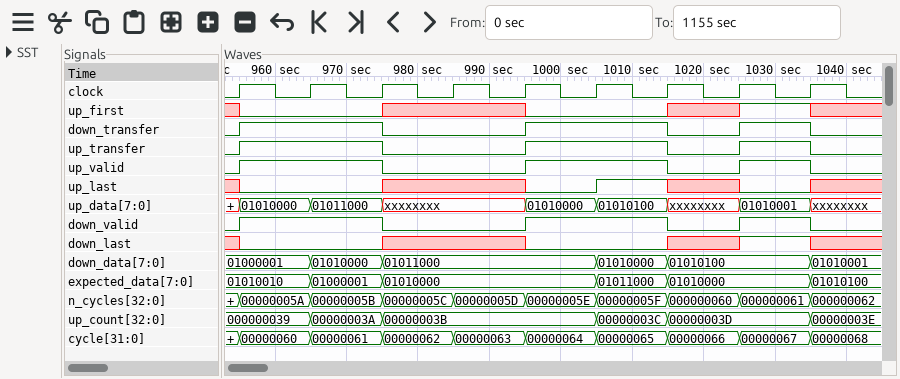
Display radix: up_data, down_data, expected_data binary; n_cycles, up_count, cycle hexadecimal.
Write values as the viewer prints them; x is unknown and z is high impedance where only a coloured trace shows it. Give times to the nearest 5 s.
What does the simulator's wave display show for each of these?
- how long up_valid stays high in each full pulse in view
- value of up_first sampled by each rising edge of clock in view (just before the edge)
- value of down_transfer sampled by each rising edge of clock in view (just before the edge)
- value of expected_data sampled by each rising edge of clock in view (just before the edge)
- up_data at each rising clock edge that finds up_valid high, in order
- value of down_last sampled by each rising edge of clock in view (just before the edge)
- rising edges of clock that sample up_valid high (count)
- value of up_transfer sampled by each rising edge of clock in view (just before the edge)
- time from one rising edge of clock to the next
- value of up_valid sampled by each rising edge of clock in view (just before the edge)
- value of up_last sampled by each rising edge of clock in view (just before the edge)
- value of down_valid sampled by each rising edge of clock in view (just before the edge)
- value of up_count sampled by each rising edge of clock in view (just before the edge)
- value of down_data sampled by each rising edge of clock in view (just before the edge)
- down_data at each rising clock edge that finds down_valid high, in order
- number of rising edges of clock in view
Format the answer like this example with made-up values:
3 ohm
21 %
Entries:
20 s, 20 s, 10 s
x 0 0 x x 0 0 x 1
0 1 1 0 0 1 1 0 1
01010010, 01010010, 01000001, 01010000, 01010000, 01010000, 01011000, 01010000, 01010000
01010000, 01011000, 01010000, 01010100, 01010001
x 0 0 x x 0 0 x 1
5
0 1 1 0 0 1 1 0 1
10 s
0 1 1 0 0 1 1 0 1
x 0 0 x x 0 1 x 0
0 1 1 0 0 1 1 0 1
000000039, 000000039, 00000003A, 00000003B, 00000003B, 00000003B, 00000003C, 00000003D, 00000003D
01000001, 01000001, 01010000, 01011000, 01011000, 01011000, 01010000, 01010100, 01010100
01000001, 01010000, 01011000, 01010000, 01010100
9
